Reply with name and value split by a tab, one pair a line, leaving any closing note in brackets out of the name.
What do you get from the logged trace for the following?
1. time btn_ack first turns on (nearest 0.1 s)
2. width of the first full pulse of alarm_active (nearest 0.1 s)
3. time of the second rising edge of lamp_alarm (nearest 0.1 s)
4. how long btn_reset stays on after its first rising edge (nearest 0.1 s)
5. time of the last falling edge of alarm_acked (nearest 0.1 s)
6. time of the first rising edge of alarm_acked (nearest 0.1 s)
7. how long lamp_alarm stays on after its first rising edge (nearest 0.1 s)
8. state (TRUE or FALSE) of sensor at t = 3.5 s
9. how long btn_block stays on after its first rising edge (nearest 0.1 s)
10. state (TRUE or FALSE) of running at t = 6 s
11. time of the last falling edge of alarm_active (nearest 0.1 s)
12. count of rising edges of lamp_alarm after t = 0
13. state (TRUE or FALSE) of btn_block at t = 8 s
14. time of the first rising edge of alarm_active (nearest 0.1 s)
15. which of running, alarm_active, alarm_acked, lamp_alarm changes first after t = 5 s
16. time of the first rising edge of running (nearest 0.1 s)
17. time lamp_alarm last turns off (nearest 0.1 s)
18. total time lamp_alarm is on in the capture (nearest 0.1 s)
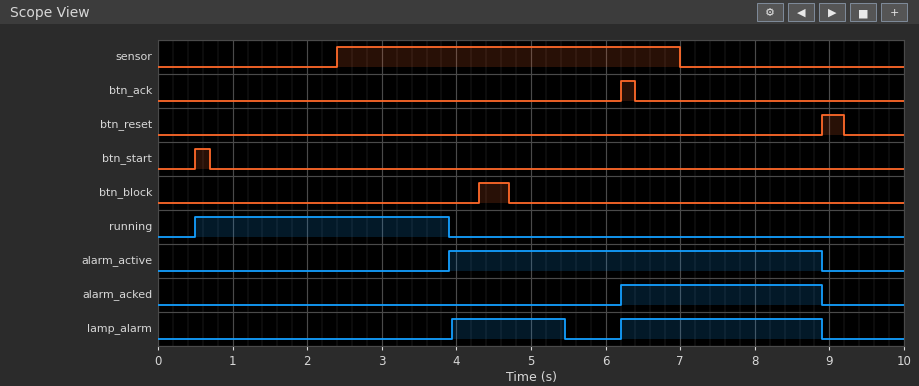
time btn_ack first turns on	6.2 s
width of the first full pulse of alarm_active	5.0 s
time of the second rising edge of lamp_alarm	6.2 s
how long btn_reset stays on after its first rising edge	0.3 s
time of the last falling edge of alarm_acked	8.9 s
time of the first rising edge of alarm_acked	6.2 s
how long lamp_alarm stays on after its first rising edge	1.5 s
state (TRUE or FALSE) of sensor at t = 3.5 s	TRUE
how long btn_block stays on after its first rising edge	0.4 s
state (TRUE or FALSE) of running at t = 6 s	FALSE
time of the last falling edge of alarm_active	8.9 s
count of rising edges of lamp_alarm after t = 0	2
state (TRUE or FALSE) of btn_block at t = 8 s	FALSE
time of the first rising edge of alarm_active	3.9 s
which of running, alarm_active, alarm_acked, lamp_alarm changes first after t = 5 s	lamp_alarm
time of the first rising edge of running	0.5 s
time lamp_alarm last turns off	8.9 s
total time lamp_alarm is on in the capture	4.2 s
